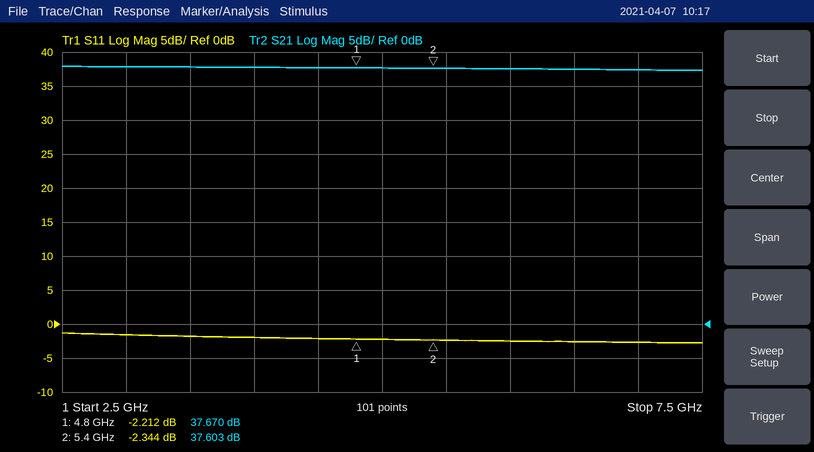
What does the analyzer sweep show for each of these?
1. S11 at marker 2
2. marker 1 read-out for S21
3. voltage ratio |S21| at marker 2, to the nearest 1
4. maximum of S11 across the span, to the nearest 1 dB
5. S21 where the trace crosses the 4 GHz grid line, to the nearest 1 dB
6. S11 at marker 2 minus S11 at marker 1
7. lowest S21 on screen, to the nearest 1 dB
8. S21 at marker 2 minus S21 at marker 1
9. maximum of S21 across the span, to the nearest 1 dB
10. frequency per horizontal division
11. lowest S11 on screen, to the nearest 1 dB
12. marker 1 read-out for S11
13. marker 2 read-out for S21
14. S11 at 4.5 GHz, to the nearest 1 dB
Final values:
-2.344 dB
37.670 dB
76
-1 dB
38 dB
-0.132 dB
37 dB
-0.067 dB
38 dB
500 MHz
-3 dB
-2.212 dB
37.603 dB
-2 dB
